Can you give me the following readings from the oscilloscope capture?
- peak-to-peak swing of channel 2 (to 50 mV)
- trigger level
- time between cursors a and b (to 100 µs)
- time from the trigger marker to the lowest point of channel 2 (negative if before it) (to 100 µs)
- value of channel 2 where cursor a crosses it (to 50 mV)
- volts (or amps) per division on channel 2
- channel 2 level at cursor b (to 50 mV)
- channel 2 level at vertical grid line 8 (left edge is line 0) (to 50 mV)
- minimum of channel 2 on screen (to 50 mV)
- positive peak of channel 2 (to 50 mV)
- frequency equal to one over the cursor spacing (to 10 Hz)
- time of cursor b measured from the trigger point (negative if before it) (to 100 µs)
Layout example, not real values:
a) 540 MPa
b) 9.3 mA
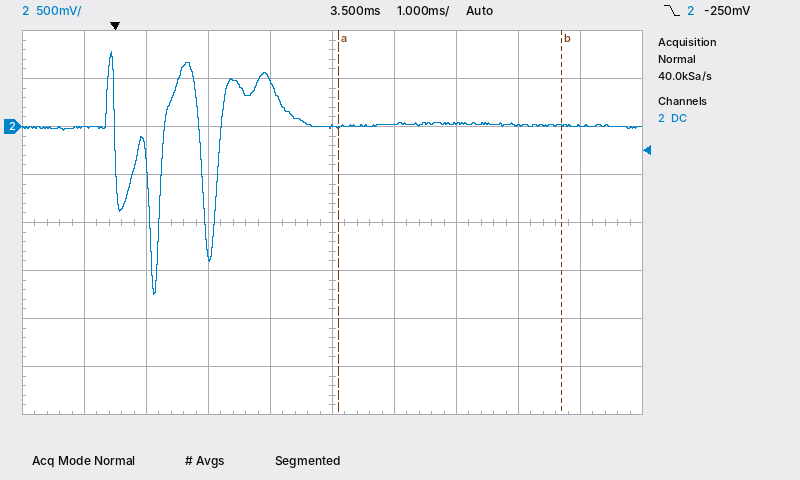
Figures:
a) 2.55 V
b) -250 mV
c) 3.6 ms
d) +600 µs
e) 0 mV
f) 500 mV
g) 0 mV
h) 0 mV
i) -1.75 V
j) 800 mV
k) 280 Hz
l) +7.2 ms
